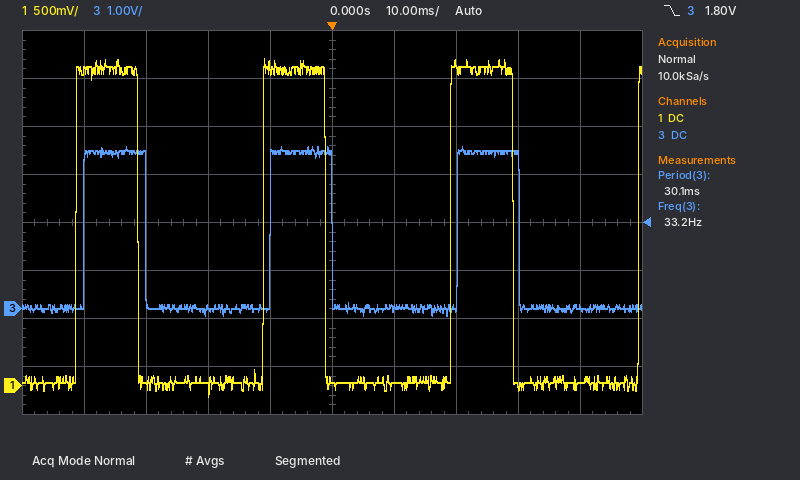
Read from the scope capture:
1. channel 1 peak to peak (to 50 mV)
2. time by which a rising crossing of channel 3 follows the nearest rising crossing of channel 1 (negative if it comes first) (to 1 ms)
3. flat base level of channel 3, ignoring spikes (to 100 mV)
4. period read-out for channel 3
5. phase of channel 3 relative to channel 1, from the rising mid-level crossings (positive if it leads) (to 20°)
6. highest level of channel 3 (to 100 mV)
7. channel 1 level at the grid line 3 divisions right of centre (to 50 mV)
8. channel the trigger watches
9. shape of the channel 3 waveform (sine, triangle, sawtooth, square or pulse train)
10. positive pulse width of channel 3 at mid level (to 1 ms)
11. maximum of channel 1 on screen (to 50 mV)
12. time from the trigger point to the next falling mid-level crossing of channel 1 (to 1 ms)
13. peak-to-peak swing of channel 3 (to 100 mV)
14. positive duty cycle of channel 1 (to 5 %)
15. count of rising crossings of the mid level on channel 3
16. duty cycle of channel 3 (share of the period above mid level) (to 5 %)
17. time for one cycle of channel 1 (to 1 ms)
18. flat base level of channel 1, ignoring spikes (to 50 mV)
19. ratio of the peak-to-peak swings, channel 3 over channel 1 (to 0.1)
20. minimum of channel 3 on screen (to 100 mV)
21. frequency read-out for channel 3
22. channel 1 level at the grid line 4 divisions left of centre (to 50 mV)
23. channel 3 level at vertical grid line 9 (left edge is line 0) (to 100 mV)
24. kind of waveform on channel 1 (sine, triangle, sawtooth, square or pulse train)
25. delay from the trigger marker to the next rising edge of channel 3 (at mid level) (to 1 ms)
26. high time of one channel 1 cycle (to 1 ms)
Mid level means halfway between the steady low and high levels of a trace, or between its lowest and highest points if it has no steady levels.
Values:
3.50 V
+1 ms
0.0 V
30.1 ms
-20°
3.4 V
0 mV
channel 3
pulse train
10 ms
3.40 V
29 ms
3.5 V
35 %
3
35 %
30 ms
50 mV
1.0
-100 mV
33.2 Hz
3.30 V
0.0 V
pulse train
20 ms
10 ms
